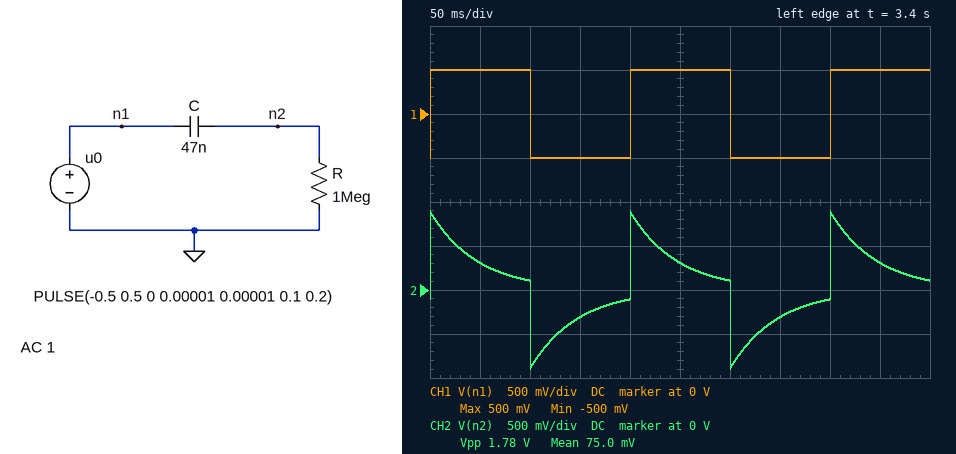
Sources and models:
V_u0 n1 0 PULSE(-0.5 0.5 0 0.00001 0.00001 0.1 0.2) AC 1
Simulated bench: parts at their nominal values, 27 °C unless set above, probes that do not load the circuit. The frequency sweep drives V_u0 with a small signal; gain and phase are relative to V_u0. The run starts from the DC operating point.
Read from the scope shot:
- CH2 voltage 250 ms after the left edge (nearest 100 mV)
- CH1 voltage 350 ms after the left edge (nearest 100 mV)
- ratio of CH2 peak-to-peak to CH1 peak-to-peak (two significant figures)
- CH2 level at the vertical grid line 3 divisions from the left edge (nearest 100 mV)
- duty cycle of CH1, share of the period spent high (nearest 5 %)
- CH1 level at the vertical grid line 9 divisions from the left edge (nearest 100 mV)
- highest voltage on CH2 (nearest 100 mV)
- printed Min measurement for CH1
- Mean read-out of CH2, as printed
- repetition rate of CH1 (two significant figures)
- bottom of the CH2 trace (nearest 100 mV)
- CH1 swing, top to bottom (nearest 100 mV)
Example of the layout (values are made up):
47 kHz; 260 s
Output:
300 mV; -500 mV; 1.8; -300 mV; 50 %; 500 mV; 900 mV; -500 mV; 75.0 mV; 5.0 Hz; -900 mV; 1.0 V
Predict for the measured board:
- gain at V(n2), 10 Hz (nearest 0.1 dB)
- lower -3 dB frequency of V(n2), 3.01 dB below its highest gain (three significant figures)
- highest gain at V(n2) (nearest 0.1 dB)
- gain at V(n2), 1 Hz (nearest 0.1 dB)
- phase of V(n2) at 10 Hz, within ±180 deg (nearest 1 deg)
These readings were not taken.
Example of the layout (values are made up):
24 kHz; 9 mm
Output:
-0.5 dB; 3.39 Hz; 0 dB; -11.0 dB; 19 deg
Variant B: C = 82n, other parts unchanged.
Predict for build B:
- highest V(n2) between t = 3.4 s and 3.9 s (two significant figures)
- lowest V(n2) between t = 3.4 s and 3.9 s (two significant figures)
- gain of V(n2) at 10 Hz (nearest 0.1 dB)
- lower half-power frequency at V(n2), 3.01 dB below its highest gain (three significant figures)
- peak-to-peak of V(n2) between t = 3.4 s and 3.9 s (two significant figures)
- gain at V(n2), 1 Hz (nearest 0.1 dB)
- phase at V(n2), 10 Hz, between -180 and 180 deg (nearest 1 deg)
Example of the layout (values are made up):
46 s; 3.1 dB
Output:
770 mV; -770 mV; -0.2 dB; 1.94 Hz; 1.5 V; -6.8 dB; 11 deg
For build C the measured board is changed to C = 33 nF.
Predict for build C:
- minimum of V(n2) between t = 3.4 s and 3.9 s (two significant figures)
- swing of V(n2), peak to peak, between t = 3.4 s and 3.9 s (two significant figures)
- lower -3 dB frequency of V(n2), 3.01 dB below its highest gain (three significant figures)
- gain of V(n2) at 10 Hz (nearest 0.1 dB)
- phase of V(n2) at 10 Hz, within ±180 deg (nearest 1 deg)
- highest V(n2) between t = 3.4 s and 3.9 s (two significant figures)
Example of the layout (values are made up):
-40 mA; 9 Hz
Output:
-950 mV; 1.9 V; 4.82 Hz; -0.9 dB; 26 deg; 950 mV
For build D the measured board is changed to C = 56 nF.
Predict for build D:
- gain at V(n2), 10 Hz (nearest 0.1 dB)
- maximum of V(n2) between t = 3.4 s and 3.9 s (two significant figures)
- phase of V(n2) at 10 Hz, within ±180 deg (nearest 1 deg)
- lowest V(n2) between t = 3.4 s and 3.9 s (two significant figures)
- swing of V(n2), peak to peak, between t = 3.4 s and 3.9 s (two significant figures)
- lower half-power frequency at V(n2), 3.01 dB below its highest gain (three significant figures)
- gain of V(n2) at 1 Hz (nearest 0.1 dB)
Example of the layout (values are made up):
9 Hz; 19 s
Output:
-0.3 dB; 860 mV; 16 deg; -860 mV; 1.7 V; 2.84 Hz; -9.6 dB
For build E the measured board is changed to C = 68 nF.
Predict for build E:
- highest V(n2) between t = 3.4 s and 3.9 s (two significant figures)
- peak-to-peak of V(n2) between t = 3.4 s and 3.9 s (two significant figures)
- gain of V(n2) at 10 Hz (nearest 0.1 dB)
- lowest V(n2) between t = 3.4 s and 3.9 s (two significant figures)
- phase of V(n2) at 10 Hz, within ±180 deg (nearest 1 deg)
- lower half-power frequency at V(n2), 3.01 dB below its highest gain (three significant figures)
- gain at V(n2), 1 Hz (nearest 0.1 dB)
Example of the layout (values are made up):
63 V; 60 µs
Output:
810 mV; 1.6 V; -0.2 dB; -810 mV; 13 deg; 2.34 Hz; -8.1 dB
